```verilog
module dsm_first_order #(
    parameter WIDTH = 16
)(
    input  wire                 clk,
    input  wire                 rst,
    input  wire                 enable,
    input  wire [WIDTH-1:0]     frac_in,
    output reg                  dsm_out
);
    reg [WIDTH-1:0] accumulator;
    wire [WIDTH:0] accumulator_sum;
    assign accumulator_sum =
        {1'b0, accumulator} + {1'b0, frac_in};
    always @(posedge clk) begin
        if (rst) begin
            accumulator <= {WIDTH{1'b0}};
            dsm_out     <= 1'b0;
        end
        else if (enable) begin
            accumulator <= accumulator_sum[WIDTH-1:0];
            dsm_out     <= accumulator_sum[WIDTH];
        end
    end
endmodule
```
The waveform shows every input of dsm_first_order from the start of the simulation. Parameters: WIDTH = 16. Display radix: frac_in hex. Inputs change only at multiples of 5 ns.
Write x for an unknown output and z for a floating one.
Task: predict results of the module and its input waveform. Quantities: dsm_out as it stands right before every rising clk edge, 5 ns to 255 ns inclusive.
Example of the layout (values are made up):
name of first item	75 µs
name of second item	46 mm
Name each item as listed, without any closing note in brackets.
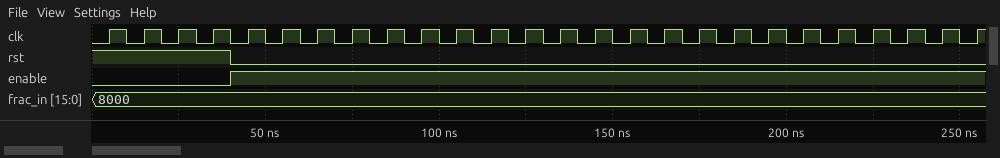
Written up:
dsm_out as it stands right before every rising clk edge, 5 ns to 255 ns inclusive	x 0 0 0 0 0 1 0 1 0 1 0 1 0 1 0 1 0 1 0 1 0 1 0 1 0
